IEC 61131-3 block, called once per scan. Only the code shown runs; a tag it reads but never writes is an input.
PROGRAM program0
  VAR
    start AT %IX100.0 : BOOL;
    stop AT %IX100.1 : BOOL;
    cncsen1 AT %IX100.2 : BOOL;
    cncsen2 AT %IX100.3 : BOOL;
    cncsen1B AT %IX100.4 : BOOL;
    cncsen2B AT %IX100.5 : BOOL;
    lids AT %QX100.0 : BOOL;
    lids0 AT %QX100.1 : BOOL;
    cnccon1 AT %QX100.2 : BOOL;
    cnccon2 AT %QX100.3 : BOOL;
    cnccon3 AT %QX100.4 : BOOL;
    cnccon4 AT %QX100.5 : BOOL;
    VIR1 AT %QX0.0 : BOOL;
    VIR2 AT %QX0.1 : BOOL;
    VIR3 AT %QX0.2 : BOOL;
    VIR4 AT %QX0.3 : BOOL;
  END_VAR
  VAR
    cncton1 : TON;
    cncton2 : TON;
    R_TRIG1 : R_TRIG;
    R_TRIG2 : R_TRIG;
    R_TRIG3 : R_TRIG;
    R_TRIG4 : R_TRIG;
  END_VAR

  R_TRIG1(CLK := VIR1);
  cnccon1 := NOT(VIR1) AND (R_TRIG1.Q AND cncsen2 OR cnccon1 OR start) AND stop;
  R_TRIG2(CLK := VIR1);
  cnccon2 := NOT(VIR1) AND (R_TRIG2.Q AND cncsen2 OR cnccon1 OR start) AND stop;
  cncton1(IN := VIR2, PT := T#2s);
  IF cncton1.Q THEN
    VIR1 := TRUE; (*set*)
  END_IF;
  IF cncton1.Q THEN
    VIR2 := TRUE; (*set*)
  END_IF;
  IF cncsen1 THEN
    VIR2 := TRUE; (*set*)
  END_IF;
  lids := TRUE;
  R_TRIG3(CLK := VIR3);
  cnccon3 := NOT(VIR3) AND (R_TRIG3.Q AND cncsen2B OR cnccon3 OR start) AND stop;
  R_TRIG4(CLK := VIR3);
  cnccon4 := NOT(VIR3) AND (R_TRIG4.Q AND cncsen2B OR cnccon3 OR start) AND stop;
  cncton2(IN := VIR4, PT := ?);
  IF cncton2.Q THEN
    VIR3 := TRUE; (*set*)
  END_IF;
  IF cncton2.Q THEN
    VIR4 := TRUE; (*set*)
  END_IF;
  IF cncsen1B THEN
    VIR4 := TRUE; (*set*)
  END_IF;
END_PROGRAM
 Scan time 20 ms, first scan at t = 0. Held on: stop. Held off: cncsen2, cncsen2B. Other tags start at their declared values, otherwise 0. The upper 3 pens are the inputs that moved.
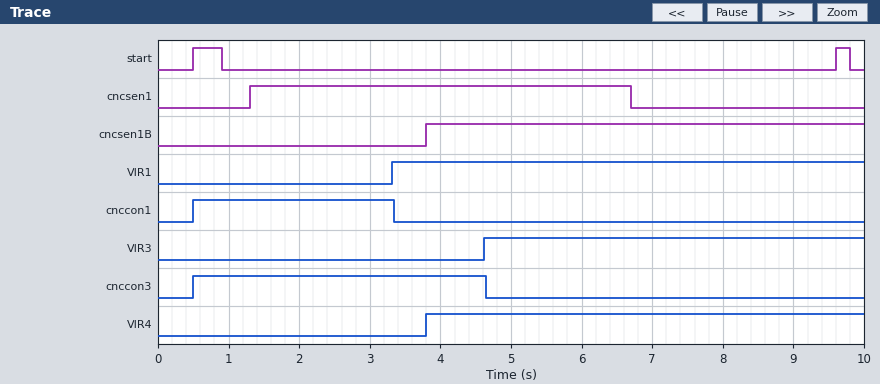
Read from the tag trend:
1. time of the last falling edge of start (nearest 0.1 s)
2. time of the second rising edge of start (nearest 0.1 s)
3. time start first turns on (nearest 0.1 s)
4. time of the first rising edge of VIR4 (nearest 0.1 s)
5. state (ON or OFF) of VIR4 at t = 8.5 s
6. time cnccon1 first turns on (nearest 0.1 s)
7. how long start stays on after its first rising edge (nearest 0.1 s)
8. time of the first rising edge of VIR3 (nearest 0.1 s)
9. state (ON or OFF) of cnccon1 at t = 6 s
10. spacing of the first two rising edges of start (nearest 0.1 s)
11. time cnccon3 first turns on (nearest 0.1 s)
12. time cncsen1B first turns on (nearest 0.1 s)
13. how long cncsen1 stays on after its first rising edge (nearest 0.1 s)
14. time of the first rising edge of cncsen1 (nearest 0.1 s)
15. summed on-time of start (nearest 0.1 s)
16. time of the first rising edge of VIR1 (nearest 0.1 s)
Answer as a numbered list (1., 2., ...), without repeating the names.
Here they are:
1. 9.8 s
2. 9.6 s
3. 0.5 s
4. 3.8 s
5. ON
6. 0.5 s
7. 0.4 s
8. 4.6 s
9. OFF
10. 9.1 s
11. 0.5 s
12. 3.8 s
13. 5.4 s
14. 1.3 s
15. 0.6 s
16. 3.3 s
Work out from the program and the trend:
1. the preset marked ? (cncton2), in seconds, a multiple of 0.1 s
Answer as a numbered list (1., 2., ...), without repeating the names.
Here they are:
1. 0.8 s
